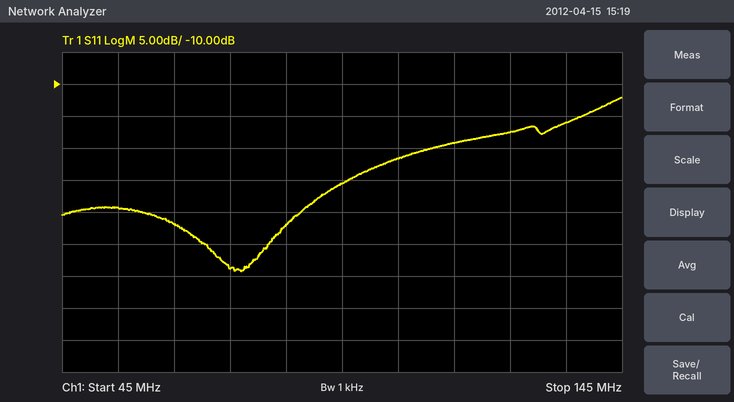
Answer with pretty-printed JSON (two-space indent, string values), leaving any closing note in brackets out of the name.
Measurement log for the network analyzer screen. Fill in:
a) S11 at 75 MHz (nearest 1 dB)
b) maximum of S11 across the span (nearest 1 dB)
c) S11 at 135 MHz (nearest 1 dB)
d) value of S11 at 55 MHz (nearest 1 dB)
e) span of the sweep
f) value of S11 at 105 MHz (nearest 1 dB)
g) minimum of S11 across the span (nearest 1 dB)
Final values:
{
  "S11 at 75 MHz": "-39 dB",
  "maximum of S11 across the span": "-12 dB",
  "S11 at 135 MHz": "-16 dB",
  "value of S11 at 55 MHz": "-29 dB",
  "span of the sweep": "100 MHz",
  "value of S11 at 105 MHz": "-22 dB",
  "minimum of S11 across the span": "-39 dB"
}
